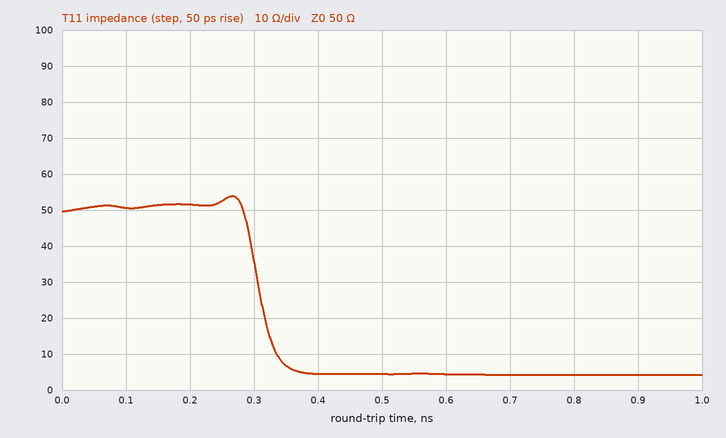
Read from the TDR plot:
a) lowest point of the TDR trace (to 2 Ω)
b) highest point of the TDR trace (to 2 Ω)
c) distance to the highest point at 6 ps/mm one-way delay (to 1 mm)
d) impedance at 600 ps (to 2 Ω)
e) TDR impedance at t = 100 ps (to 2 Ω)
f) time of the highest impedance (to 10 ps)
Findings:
4 Ω
54 Ω
22 mm
4 Ω
50 Ω
270 ps
